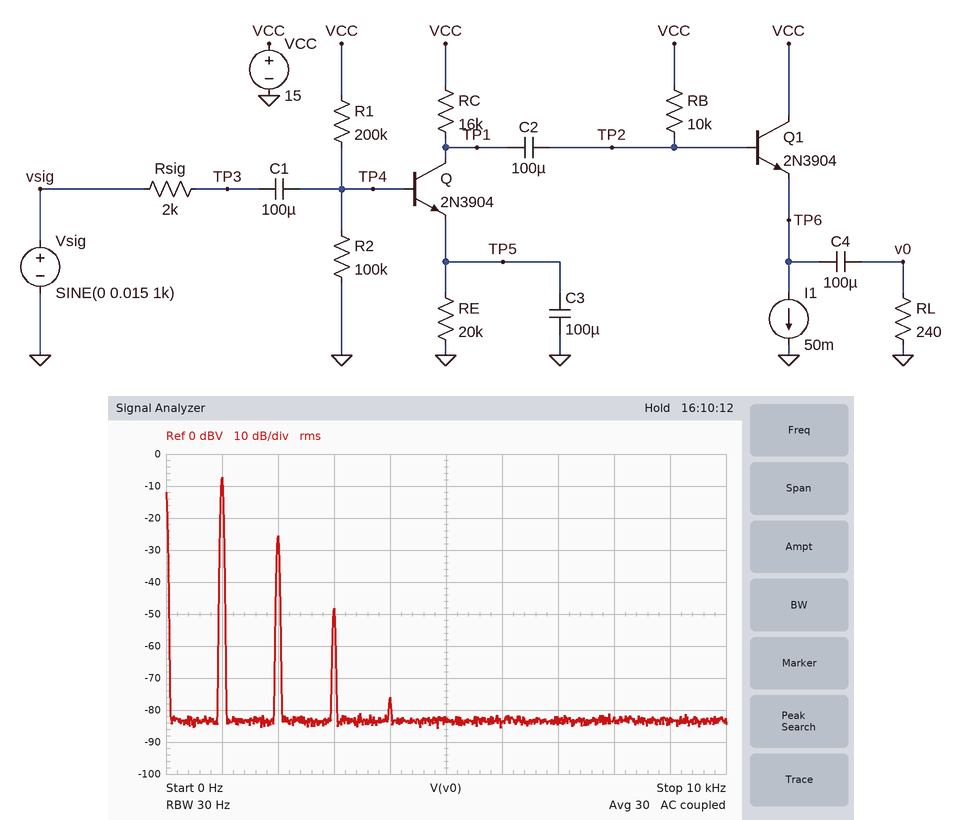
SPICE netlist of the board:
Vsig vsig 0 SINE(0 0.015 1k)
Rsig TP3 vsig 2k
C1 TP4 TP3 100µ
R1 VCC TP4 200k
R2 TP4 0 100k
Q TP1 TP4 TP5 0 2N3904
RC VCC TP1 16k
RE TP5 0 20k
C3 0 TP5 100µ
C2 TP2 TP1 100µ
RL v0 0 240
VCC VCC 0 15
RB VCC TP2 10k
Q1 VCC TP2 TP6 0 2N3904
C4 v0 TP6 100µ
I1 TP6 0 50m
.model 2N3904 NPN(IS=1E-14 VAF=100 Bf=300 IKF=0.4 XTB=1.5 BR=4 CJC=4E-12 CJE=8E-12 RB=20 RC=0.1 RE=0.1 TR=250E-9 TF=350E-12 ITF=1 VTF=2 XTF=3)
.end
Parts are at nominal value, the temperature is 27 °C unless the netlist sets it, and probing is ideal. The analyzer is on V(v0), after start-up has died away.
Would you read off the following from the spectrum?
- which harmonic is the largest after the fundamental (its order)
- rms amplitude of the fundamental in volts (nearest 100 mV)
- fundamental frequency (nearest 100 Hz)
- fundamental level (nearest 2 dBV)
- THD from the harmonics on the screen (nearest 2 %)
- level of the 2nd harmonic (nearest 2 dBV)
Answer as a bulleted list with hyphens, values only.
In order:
- 2
- 400 mV
- 1.0 kHz
- -8 dBV
- 12 %
- -26 dBV
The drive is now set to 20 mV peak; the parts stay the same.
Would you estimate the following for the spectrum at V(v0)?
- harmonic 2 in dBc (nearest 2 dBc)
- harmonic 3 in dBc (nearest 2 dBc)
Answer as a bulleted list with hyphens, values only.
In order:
- -16 dBc
- -36 dBc
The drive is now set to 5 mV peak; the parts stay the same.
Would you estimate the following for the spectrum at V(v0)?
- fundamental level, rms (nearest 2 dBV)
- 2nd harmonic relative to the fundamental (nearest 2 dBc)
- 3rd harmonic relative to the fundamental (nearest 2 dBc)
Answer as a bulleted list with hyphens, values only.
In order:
- -16 dBV
- -28 dBc
- -60 dBc
